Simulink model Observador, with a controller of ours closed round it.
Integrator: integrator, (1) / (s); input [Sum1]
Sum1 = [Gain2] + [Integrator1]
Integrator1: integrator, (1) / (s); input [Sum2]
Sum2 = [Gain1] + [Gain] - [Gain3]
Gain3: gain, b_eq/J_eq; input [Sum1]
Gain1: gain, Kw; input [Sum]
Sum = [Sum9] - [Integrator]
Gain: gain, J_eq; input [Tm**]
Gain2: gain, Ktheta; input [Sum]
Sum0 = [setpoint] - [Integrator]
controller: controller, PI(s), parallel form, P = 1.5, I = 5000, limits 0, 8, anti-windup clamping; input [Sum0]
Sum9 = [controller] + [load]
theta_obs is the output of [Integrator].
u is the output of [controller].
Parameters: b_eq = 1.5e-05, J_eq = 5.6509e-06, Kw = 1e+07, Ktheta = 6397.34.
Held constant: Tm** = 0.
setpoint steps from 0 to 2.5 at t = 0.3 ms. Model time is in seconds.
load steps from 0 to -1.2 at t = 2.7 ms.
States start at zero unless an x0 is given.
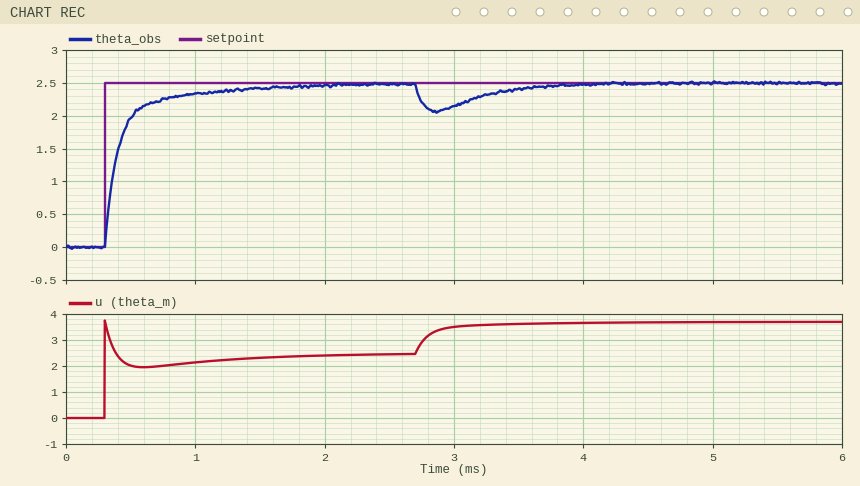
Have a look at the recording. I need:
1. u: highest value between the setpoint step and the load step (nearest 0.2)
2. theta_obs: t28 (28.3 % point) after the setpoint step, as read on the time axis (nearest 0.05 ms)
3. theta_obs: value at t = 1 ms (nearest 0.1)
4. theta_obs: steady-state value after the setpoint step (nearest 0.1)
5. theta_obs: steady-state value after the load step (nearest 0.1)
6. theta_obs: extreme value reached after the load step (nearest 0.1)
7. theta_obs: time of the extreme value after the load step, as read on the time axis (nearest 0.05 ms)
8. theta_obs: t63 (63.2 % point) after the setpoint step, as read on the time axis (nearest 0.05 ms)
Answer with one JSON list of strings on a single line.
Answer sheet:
["3.8", "0.35 ms", "2.3", "2.5", "2.5", "2.1", "2.85 ms", "0.40 ms"]
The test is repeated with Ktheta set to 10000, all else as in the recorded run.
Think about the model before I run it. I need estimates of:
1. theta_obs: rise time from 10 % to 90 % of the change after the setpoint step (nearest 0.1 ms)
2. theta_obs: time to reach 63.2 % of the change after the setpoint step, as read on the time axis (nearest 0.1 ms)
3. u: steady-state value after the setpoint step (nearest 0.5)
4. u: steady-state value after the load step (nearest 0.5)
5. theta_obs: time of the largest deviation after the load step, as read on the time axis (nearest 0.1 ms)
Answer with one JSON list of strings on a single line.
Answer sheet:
["0.6 ms", "0.4 ms", "2.5", "3.5", "2.8 ms"]
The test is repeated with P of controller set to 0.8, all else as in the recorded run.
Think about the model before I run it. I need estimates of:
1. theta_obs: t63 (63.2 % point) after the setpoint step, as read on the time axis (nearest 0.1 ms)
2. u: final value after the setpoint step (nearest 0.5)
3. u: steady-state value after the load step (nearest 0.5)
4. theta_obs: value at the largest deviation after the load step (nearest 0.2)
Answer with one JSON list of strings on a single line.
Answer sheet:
["0.5 ms", "2.5", "3.5", "2.0"]
